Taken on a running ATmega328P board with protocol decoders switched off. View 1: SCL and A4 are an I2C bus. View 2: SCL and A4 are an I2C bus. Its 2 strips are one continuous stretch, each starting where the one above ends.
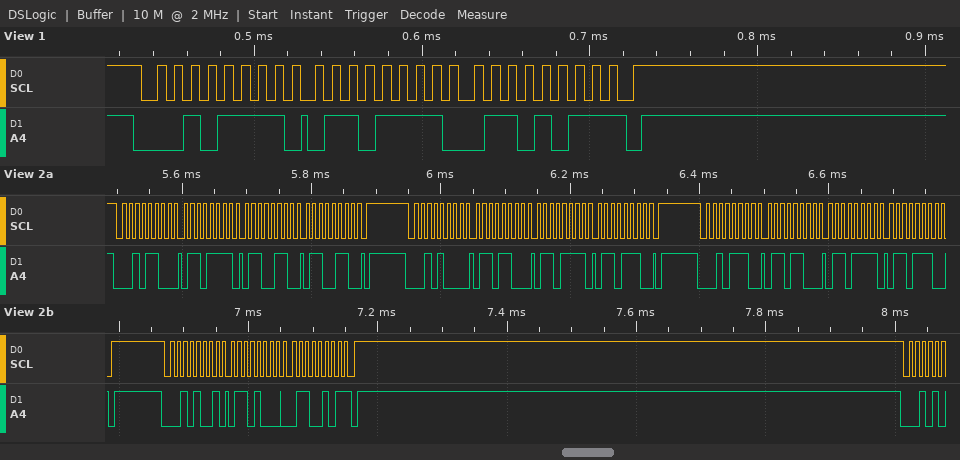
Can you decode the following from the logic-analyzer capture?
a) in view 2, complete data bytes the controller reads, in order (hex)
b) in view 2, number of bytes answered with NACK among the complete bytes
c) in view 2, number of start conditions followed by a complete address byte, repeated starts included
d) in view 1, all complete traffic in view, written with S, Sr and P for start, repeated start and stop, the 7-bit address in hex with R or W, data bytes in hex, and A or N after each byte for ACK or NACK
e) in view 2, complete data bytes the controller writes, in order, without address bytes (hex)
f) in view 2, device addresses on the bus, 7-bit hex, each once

68 65
1
4
S 17R A 6F A 6B N P
6F 66 66 6C 6F 6E 6C 6F 6E
0x16 0x14 0x17
